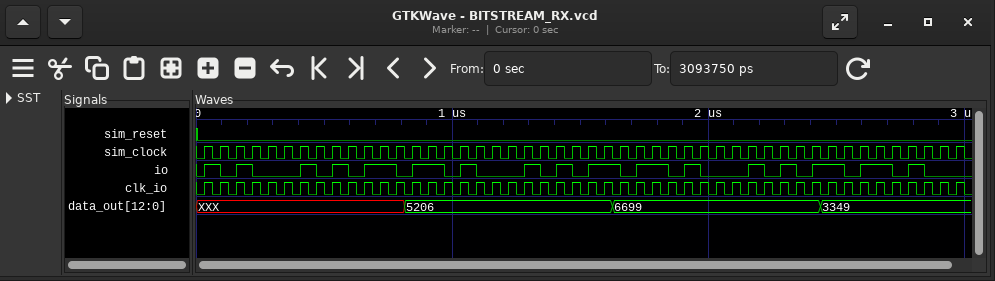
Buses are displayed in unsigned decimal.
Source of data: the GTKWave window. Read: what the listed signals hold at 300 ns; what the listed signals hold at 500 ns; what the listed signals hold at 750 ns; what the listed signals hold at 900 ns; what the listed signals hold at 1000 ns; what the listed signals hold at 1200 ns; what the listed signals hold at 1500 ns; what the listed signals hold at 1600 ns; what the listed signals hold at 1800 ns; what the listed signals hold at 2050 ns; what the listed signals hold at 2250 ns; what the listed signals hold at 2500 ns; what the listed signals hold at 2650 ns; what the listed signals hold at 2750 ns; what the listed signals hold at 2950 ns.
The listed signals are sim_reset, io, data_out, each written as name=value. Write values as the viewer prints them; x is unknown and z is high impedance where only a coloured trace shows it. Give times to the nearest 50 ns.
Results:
sim_reset=0, io=0, data_out=XXX
sim_reset=0, io=0, data_out=XXX
sim_reset=0, io=1, data_out=XXX
sim_reset=0, io=1, data_out=5206
sim_reset=0, io=0, data_out=5206
sim_reset=0, io=0, data_out=5206
sim_reset=0, io=0, data_out=5206
sim_reset=0, io=1, data_out=5206
sim_reset=0, io=1, data_out=6699
sim_reset=0, io=0, data_out=6699
sim_reset=0, io=0, data_out=6699
sim_reset=0, io=1, data_out=3349
sim_reset=0, io=1, data_out=3349
sim_reset=0, io=0, data_out=3349
sim_reset=0, io=0, data_out=3349
